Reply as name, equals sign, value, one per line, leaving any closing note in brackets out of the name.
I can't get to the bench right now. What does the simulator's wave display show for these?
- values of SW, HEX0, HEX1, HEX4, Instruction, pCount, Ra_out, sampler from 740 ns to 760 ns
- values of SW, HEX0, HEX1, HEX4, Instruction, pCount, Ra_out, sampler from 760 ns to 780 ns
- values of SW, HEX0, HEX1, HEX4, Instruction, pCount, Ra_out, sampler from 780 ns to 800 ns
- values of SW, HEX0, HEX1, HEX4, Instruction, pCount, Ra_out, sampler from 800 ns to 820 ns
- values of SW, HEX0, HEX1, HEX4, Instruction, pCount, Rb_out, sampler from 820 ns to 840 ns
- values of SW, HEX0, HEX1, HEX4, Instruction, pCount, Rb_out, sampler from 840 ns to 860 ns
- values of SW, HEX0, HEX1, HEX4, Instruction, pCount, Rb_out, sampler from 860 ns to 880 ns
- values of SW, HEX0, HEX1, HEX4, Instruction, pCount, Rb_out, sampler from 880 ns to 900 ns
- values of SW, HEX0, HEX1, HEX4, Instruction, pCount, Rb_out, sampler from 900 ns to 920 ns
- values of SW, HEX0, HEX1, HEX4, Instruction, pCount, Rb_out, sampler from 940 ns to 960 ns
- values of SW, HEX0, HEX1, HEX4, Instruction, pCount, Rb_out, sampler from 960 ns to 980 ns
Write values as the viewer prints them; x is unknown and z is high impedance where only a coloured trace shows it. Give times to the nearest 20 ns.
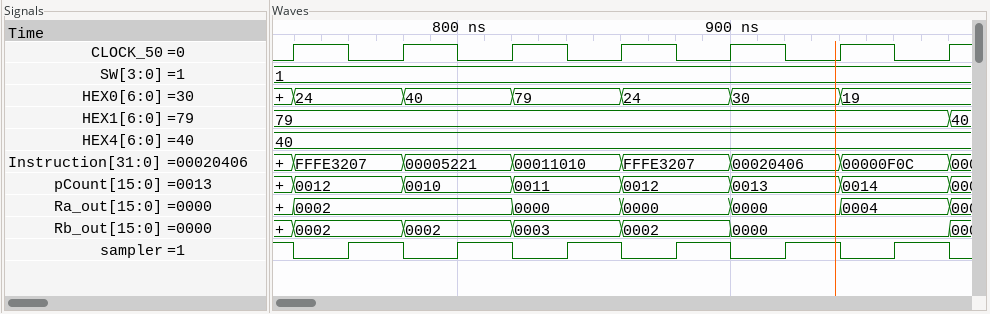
values of SW, HEX0, HEX1, HEX4, Instruction, pCount, Ra_out, sampler from 740 ns to 760 ns = SW=1, HEX0=24, HEX1=79, HEX4=40, Instruction=FFFE3207, pCount=0012, Ra_out=0002, sampler=0
values of SW, HEX0, HEX1, HEX4, Instruction, pCount, Ra_out, sampler from 760 ns to 780 ns = SW=1, HEX0=24, HEX1=79, HEX4=40, Instruction=FFFE3207, pCount=0012, Ra_out=0002, sampler=1
values of SW, HEX0, HEX1, HEX4, Instruction, pCount, Ra_out, sampler from 780 ns to 800 ns = SW=1, HEX0=40, HEX1=79, HEX4=40, Instruction=00005221, pCount=0010, Ra_out=0002, sampler=0
values of SW, HEX0, HEX1, HEX4, Instruction, pCount, Ra_out, sampler from 800 ns to 820 ns = SW=1, HEX0=40, HEX1=79, HEX4=40, Instruction=00005221, pCount=0010, Ra_out=0002, sampler=1
values of SW, HEX0, HEX1, HEX4, Instruction, pCount, Rb_out, sampler from 820 ns to 840 ns = SW=1, HEX0=79, HEX1=79, HEX4=40, Instruction=00011010, pCount=0011, Rb_out=0003, sampler=0
values of SW, HEX0, HEX1, HEX4, Instruction, pCount, Rb_out, sampler from 840 ns to 860 ns = SW=1, HEX0=79, HEX1=79, HEX4=40, Instruction=00011010, pCount=0011, Rb_out=0003, sampler=1
values of SW, HEX0, HEX1, HEX4, Instruction, pCount, Rb_out, sampler from 860 ns to 880 ns = SW=1, HEX0=24, HEX1=79, HEX4=40, Instruction=FFFE3207, pCount=0012, Rb_out=0002, sampler=0
values of SW, HEX0, HEX1, HEX4, Instruction, pCount, Rb_out, sampler from 880 ns to 900 ns = SW=1, HEX0=24, HEX1=79, HEX4=40, Instruction=FFFE3207, pCount=0012, Rb_out=0002, sampler=1
values of SW, HEX0, HEX1, HEX4, Instruction, pCount, Rb_out, sampler from 900 ns to 920 ns = SW=1, HEX0=30, HEX1=79, HEX4=40, Instruction=00020406, pCount=0013, Rb_out=0000, sampler=0
values of SW, HEX0, HEX1, HEX4, Instruction, pCount, Rb_out, sampler from 940 ns to 960 ns = SW=1, HEX0=19, HEX1=79, HEX4=40, Instruction=00000F0C, pCount=0014, Rb_out=0000, sampler=0
values of SW, HEX0, HEX1, HEX4, Instruction, pCount, Rb_out, sampler from 960 ns to 980 ns = SW=1, HEX0=19, HEX1=79, HEX4=40, Instruction=00000F0C, pCount=0014, Rb_out=0000, sampler=1
